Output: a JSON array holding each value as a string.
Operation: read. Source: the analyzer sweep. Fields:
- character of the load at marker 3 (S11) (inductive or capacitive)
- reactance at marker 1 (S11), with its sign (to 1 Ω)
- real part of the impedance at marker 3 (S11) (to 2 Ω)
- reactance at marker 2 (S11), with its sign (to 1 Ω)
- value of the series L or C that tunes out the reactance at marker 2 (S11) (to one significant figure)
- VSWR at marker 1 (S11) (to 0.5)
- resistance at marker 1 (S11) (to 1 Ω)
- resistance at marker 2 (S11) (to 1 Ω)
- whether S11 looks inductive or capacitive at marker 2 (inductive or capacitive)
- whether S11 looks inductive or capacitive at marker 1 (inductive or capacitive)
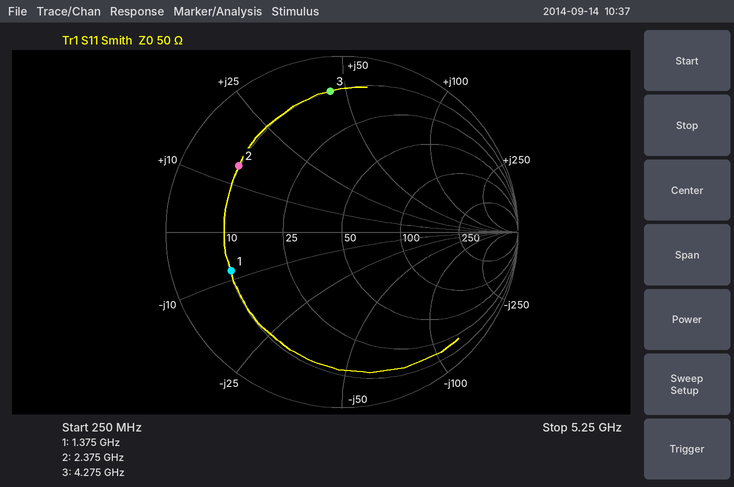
["inductive", "-8 Ω", "10 Ω", "+14 Ω", "5 pF", "5.0", "10 Ω", "10 Ω", "inductive", "capacitive"]
